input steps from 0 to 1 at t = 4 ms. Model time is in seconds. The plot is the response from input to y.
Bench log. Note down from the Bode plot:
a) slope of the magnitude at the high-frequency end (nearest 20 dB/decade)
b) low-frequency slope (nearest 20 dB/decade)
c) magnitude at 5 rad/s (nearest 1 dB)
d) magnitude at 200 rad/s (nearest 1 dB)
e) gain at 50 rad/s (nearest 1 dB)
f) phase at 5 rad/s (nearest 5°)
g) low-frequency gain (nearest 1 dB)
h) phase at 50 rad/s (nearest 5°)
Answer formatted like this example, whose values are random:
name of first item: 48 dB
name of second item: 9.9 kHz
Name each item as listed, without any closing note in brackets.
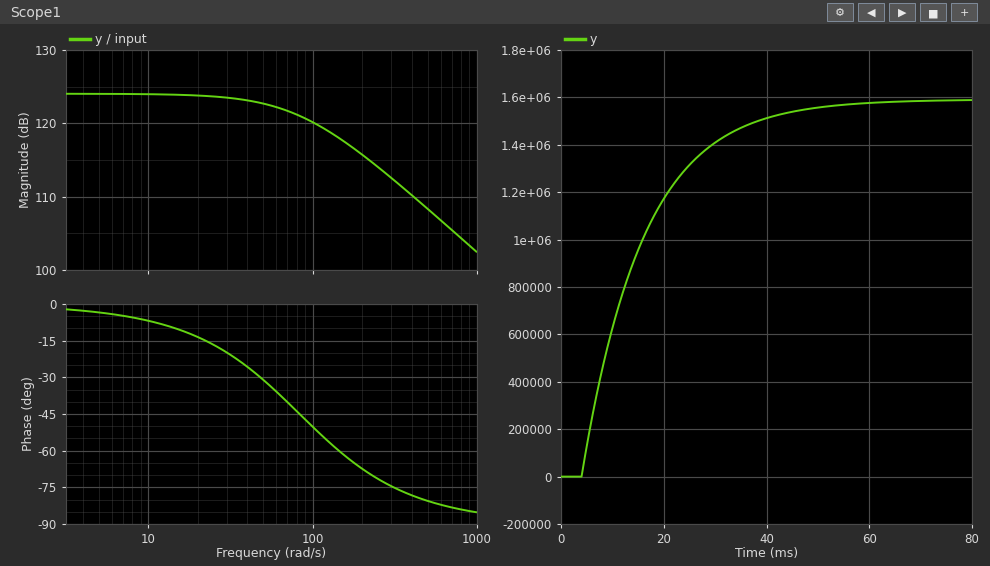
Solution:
slope of the magnitude at the high-frequency end: -20 dB/decade
low-frequency slope: 0 dB/decade
magnitude at 5 rad/s: 124 dB
magnitude at 200 rad/s: 116 dB
gain at 50 rad/s: 123 dB
phase at 5 rad/s: -5°
low-frequency gain: 124 dB
phase at 50 rad/s: -30°
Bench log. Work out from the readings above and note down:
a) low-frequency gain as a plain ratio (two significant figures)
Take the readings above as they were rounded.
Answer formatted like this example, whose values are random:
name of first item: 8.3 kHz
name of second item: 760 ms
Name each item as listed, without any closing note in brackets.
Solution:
low-frequency gain as a plain ratio: 1600000
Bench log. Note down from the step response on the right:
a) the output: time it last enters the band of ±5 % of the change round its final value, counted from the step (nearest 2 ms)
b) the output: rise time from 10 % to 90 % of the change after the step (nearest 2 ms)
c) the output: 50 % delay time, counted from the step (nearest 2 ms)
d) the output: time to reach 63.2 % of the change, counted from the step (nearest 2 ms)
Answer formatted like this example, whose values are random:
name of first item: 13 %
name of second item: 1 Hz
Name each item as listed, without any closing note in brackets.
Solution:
the output: time it last enters the band of ±5 % of the change round its final value, counted from the step: 36 ms
the output: rise time from 10 % to 90 % of the change after the step: 26 ms
the output: 50 % delay time, counted from the step: 8 ms
the output: time to reach 63.2 % of the change, counted from the step: 12 ms
